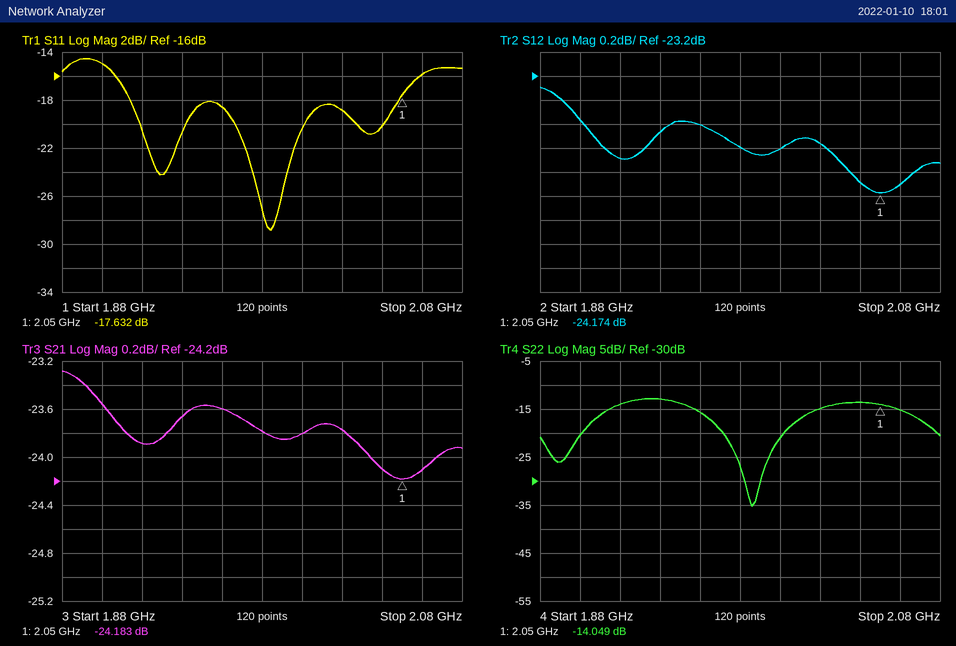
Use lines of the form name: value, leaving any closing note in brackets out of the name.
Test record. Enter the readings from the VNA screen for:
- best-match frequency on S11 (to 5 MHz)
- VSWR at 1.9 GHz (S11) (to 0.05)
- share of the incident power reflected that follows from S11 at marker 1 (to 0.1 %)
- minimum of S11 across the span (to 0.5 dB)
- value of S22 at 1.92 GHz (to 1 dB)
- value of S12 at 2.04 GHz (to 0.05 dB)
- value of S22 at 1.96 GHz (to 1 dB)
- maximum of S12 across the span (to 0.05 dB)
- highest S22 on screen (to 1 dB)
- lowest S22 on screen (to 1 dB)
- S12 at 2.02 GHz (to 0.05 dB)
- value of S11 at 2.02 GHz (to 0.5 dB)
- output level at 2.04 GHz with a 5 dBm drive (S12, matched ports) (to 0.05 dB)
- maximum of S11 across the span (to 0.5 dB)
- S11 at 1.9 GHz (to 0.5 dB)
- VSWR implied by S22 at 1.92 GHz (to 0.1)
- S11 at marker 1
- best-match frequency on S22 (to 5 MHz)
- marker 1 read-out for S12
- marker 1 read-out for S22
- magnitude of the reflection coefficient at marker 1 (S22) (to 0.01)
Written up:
best-match frequency on S11: 1.985 GHz
VSWR at 1.9 GHz (S11): 1.45
share of the incident power reflected that follows from S11 at marker 1: 1.7 %
minimum of S11 across the span: -29.0 dB
value of S22 at 1.92 GHz: -14 dB
value of S12 at 2.04 GHz: -24.10 dB
value of S22 at 1.96 GHz: -16 dB
maximum of S12 across the span: -23.30 dB
highest S22 on screen: -13 dB
lowest S22 on screen: -35 dB
S12 at 2.02 GHz: -23.75 dB
value of S11 at 2.02 GHz: -19.0 dB
output level at 2.04 GHz with a 5 dBm drive (S12, matched ports): -19.10 dBm
maximum of S11 across the span: -14.5 dB
S11 at 1.9 GHz: -15.0 dB
VSWR implied by S22 at 1.92 GHz: 1.5
S11 at marker 1: -17.632 dB
best-match frequency on S22: 1.985 GHz
marker 1 read-out for S12: -24.174 dB
marker 1 read-out for S22: -14.049 dB
magnitude of the reflection coefficient at marker 1 (S22): 0.20
